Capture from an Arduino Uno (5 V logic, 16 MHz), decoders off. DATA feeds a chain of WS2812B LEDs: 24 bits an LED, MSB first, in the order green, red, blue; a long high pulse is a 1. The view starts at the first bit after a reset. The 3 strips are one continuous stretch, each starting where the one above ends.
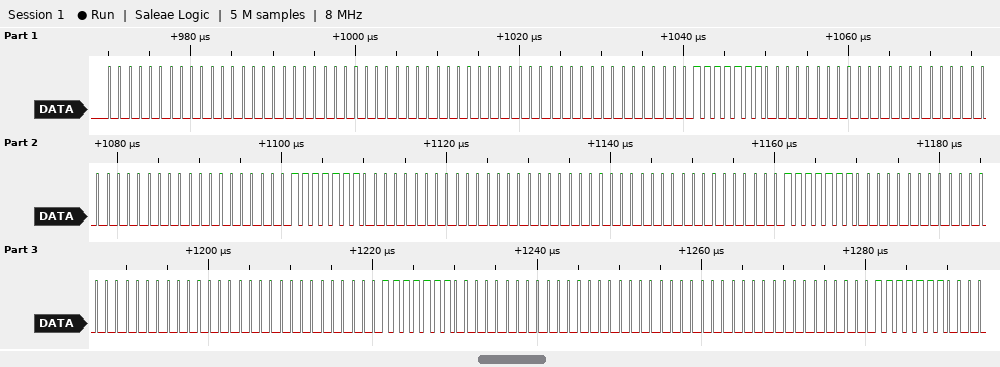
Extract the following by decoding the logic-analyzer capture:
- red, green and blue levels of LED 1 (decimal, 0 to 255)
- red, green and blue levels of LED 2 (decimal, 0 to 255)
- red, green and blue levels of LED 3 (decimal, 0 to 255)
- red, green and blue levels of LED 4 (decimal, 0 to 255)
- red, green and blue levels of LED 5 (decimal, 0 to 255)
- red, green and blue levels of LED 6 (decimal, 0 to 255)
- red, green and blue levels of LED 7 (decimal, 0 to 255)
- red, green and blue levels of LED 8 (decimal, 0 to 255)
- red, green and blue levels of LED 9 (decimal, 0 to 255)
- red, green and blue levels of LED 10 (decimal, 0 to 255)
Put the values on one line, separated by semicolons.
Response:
0, 0, 0; 0, 0, 0; 127, 0, 0; 0, 0, 0; 127, 0, 0; 0, 0, 0; 127, 0, 0; 0, 0, 0; 127, 0, 0; 0, 0, 0
